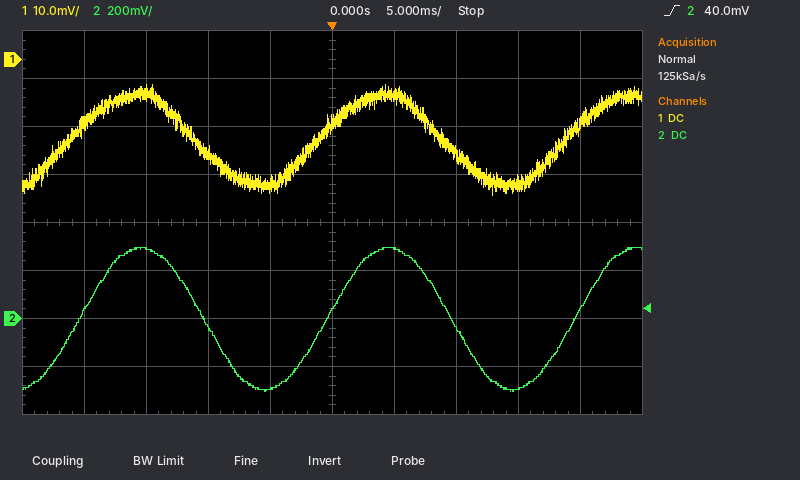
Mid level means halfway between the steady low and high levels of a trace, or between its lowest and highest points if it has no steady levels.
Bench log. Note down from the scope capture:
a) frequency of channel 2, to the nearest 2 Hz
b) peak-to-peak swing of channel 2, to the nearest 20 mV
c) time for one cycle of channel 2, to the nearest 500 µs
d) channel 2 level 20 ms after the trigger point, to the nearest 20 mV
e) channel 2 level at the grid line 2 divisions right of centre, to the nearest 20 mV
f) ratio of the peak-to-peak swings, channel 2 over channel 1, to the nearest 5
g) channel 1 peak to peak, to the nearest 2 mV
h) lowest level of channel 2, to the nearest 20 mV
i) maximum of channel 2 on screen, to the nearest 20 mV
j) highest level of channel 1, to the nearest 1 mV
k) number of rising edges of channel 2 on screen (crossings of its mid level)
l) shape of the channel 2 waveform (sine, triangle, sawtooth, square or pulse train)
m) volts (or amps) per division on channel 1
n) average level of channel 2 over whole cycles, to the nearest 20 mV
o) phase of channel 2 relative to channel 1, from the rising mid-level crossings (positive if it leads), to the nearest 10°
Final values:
50 Hz
600 mV
20.0 ms
40 mV
-40 mV
25
24 mV
-300 mV
300 mV
-5 mV
3
sine
10 mV
0 mV
-10°
